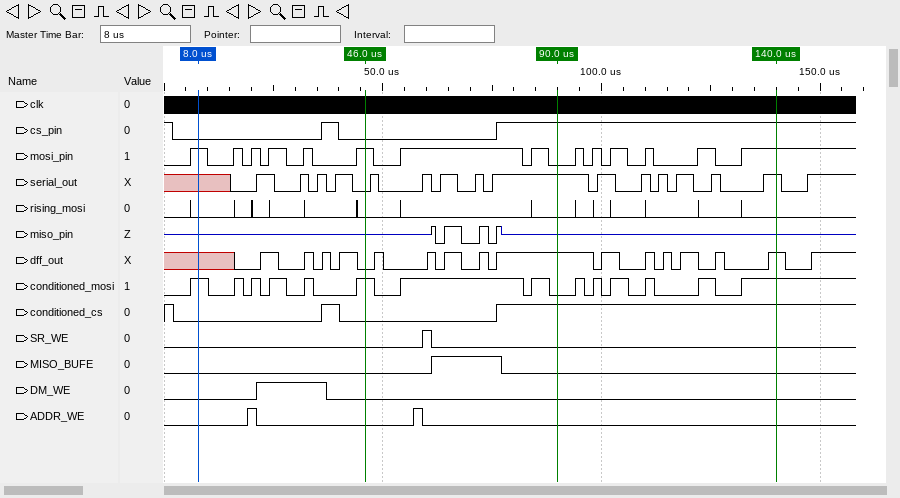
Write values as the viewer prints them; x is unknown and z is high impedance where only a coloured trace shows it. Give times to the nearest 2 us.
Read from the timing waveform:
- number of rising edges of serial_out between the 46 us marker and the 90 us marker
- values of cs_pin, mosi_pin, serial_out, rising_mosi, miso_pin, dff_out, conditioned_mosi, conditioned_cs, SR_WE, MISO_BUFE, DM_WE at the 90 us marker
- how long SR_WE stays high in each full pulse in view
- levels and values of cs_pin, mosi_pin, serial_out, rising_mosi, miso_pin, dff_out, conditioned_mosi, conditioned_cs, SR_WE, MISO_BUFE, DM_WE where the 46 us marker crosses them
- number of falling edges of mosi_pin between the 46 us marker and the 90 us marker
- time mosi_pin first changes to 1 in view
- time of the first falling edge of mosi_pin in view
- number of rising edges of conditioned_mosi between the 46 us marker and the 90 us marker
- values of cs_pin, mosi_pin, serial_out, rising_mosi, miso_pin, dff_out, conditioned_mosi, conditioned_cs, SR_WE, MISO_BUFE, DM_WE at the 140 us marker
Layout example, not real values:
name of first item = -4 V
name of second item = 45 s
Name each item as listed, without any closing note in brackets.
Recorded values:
number of rising edges of serial_out between the 46 us marker and the 90 us marker = 5
values of cs_pin, mosi_pin, serial_out, rising_mosi, miso_pin, dff_out, conditioned_mosi, conditioned_cs, SR_WE, MISO_BUFE, DM_WE at the 90 us marker = cs_pin=1, mosi_pin=0, serial_out=1, rising_mosi=0, miso_pin=z, dff_out=1, conditioned_mosi=0, conditioned_cs=1, SR_WE=0, MISO_BUFE=0, DM_WE=0
how long SR_WE stays high in each full pulse in view = 2 us
levels and values of cs_pin, mosi_pin, serial_out, rising_mosi, miso_pin, dff_out, conditioned_mosi, conditioned_cs, SR_WE, MISO_BUFE, DM_WE where the 46 us marker crosses them = cs_pin=0, mosi_pin=1, serial_out=0, rising_mosi=0, miso_pin=z, dff_out=0, conditioned_mosi=1, conditioned_cs=0, SR_WE=0, MISO_BUFE=0, DM_WE=0
number of falling edges of mosi_pin between the 46 us marker and the 90 us marker = 3
time mosi_pin first changes to 1 in view = 6 us
time of the first falling edge of mosi_pin in view = 10 us
number of rising edges of conditioned_mosi between the 46 us marker and the 90 us marker = 2
values of cs_pin, mosi_pin, serial_out, rising_mosi, miso_pin, dff_out, conditioned_mosi, conditioned_cs, SR_WE, MISO_BUFE, DM_WE at the 140 us marker = cs_pin=1, mosi_pin=1, serial_out=1, rising_mosi=0, miso_pin=z, dff_out=1, conditioned_mosi=1, conditioned_cs=1, SR_WE=0, MISO_BUFE=0, DM_WE=0
